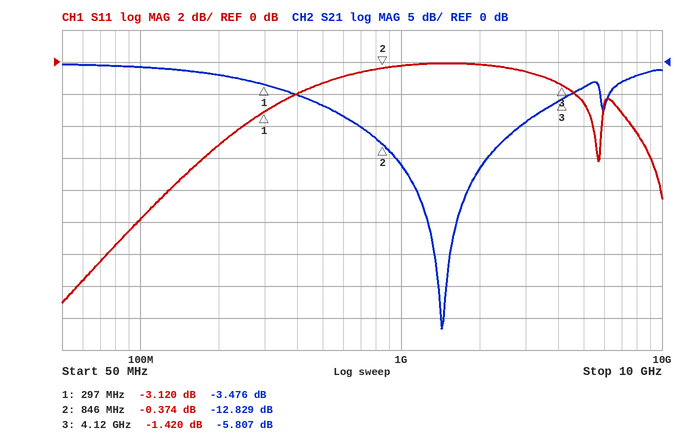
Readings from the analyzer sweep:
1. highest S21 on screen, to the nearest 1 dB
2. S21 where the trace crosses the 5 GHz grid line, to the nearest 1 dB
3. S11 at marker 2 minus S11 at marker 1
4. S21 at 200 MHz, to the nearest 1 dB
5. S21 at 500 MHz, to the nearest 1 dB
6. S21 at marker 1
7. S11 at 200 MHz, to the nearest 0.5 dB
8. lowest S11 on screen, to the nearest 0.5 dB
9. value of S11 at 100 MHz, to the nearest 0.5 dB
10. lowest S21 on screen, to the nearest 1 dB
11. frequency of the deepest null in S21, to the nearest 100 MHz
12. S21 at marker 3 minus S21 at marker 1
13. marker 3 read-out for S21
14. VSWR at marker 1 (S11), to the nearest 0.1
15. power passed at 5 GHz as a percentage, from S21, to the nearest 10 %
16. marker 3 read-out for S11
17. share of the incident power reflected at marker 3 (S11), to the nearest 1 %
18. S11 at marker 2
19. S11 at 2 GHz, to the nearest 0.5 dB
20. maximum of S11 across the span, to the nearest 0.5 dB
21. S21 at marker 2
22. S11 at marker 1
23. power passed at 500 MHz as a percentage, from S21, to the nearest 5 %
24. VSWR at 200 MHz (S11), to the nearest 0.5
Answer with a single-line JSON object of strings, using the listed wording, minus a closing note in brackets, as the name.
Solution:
{"highest S21 on screen, to the nearest 1 dB": "0 dB", "S21 where the trace crosses the 5 GHz grid line, to the nearest 1 dB": "-4 dB", "S11 at marker 2 minus S11 at marker 1": "2.746 dB", "S21 at 200 MHz, to the nearest 1 dB": "-2 dB", "S21 at 500 MHz, to the nearest 1 dB": "-7 dB", "S21 at marker 1": "-3.476 dB", "S11 at 200 MHz, to the nearest 0.5 dB": "-5.0 dB", "lowest S11 on screen, to the nearest 0.5 dB": "-15.0 dB", "value of S11 at 100 MHz, to the nearest 0.5 dB": "-10.0 dB", "lowest S21 on screen, to the nearest 1 dB": "-42 dB", "frequency of the deepest null in S21, to the nearest 100 MHz": "1.4 GHz", "S21 at marker 3 minus S21 at marker 1": "-2.331 dB", "marker 3 read-out for S21": "-5.807 dB", "VSWR at marker 1 (S11), to the nearest 0.1": "5.6", "power passed at 5 GHz as a percentage, from S21, to the nearest 10 %": "40 %", "marker 3 read-out for S11": "-1.420 dB", "share of the incident power reflected at marker 3 (S11), to the nearest 1 %": "72 %", "S11 at marker 2": "-0.374 dB", "S11 at 2 GHz, to the nearest 0.5 dB": "0.0 dB", "maximum of S11 across the span, to the nearest 0.5 dB": "0.0 dB", "S21 at marker 2": "-12.829 dB", "S11 at marker 1": "-3.120 dB", "power passed at 500 MHz as a percentage, from S21, to the nearest 5 %": "20 %", "VSWR at 200 MHz (S11), to the nearest 0.5": "3.5"}
